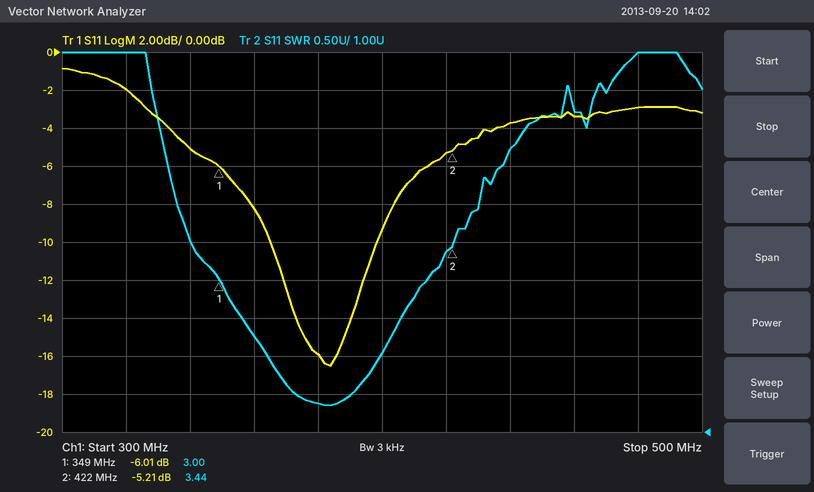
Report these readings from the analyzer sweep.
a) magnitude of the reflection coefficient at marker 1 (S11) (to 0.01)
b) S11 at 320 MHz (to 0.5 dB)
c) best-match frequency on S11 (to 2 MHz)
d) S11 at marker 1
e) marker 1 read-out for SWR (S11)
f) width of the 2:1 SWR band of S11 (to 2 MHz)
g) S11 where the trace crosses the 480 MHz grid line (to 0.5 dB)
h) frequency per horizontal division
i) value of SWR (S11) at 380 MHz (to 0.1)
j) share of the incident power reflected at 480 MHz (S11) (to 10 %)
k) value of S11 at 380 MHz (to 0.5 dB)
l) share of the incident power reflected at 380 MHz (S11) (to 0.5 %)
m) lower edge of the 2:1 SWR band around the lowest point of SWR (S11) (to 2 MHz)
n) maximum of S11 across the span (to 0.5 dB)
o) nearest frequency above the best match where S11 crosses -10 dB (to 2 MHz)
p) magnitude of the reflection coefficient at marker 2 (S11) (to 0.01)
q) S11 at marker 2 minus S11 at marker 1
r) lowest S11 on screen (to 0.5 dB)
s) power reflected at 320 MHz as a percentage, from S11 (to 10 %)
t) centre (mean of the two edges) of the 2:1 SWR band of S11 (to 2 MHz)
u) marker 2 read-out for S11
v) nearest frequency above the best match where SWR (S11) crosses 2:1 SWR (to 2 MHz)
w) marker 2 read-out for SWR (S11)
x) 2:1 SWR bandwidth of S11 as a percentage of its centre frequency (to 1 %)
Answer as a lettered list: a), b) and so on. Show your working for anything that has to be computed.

a) 10^(-6.01/20) ≈ 0.50
b) -2.0 dB
c) 384 MHz
d) -6.01 dB
e) 3.00
f) 400 MHz − 364 MHz = 36 MHz
g) -3.0 dB
h) 20 MHz
i) 1.4
j) 10^(-3/10) ≈ 50 %
k) -16.0 dB
l) 10^(-16/10) ≈ 2.5 %
m) 364 MHz
n) -1.0 dB
o) 398 MHz
p) 10^(-5.21/20) ≈ 0.55
q) -5.21 − (-6.01) = 0.80 dB
r) -16.5 dB
s) 10^(-2/10) ≈ 63.1 %, so 60 % to the nearest 10 %
t) 382 MHz
u) -5.21 dB
v) 400 MHz
w) 3.44
x) 36 MHz / 382 MHz ≈ 9 %
